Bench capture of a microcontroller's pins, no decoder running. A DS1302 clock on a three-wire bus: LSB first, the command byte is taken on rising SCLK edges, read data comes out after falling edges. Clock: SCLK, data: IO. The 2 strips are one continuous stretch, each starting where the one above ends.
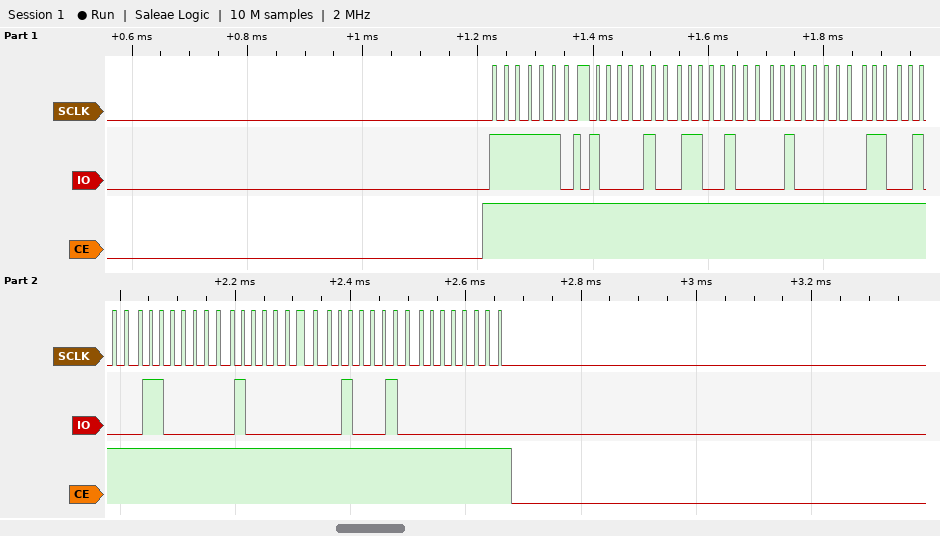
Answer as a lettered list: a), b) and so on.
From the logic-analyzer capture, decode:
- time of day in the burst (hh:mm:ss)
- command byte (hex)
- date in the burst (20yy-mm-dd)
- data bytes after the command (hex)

a) 02:13:21
b) 0xBF
c) 2022-03-13
d) 21 13 02 13 03 01 22 00
